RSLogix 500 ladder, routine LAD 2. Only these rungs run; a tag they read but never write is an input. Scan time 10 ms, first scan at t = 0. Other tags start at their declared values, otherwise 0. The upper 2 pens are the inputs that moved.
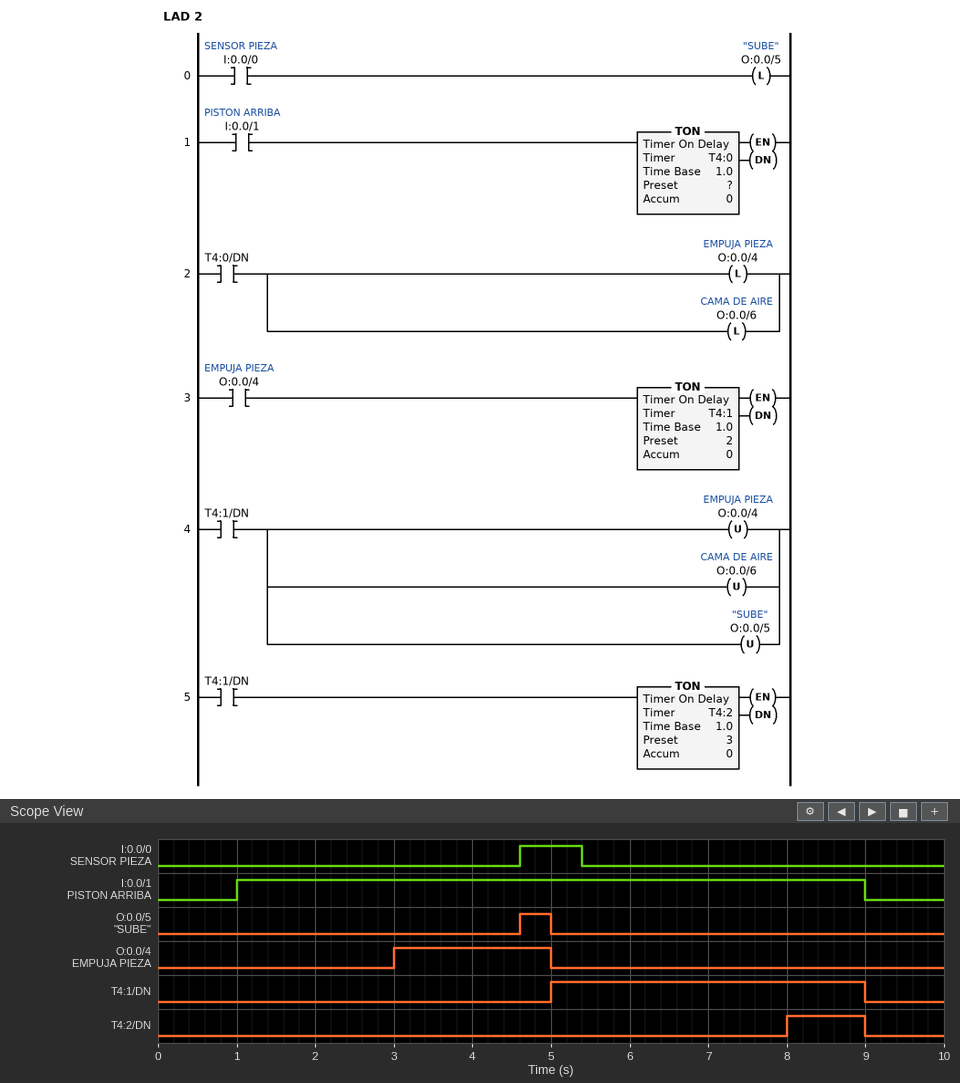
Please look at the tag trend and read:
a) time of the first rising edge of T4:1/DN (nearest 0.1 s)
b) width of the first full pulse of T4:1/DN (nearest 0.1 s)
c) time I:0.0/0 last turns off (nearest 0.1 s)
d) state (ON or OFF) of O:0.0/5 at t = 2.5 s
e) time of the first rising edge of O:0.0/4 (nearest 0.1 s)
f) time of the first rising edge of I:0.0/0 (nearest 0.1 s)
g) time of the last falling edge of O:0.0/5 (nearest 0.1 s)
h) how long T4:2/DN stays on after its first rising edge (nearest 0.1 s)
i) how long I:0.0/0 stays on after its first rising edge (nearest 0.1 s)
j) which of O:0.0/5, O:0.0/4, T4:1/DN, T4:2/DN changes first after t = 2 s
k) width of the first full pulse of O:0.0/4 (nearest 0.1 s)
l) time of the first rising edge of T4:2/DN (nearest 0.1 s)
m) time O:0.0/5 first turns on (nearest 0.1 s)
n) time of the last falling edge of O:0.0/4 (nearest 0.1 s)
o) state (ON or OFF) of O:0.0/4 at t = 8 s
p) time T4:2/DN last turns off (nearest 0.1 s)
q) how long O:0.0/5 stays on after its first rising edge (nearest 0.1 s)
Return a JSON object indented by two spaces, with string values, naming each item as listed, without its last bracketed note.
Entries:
{
  "time of the first rising edge of T4:1/DN": "5.0 s",
  "width of the first full pulse of T4:1/DN": "4.0 s",
  "time I:0.0/0 last turns off": "5.4 s",
  "state (ON or OFF) of O:0.0/5 at t = 2.5 s": "OFF",
  "time of the first rising edge of O:0.0/4": "3.0 s",
  "time of the first rising edge of I:0.0/0": "4.6 s",
  "time of the last falling edge of O:0.0/5": "5.0 s",
  "how long T4:2/DN stays on after its first rising edge": "1.0 s",
  "how long I:0.0/0 stays on after its first rising edge": "0.8 s",
  "which of O:0.0/5, O:0.0/4, T4:1/DN, T4:2/DN changes first after t = 2 s": "O:0.0/4",
  "width of the first full pulse of O:0.0/4": "2.0 s",
  "time of the first rising edge of T4:2/DN": "8.0 s",
  "time O:0.0/5 first turns on": "4.6 s",
  "time of the last falling edge of O:0.0/4": "5.0 s",
  "state (ON or OFF) of O:0.0/4 at t = 8 s": "OFF",
  "time T4:2/DN last turns off": "9.0 s",
  "how long O:0.0/5 stays on after its first rising edge": "0.4 s"
}
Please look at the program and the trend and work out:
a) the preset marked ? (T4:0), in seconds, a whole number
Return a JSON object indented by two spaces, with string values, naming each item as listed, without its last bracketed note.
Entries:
{
  "the preset marked ? (T4:0), in seconds, a whole number": "2 s"
}
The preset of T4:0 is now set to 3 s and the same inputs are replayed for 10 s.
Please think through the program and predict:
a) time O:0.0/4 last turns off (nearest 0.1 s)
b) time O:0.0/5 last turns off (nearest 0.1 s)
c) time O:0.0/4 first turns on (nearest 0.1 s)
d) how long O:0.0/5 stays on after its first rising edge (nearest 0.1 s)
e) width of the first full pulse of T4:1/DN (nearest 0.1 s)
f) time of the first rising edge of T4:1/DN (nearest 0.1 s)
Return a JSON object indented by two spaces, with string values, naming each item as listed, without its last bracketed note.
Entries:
{
  "time O:0.0/4 last turns off": "6.0 s",
  "time O:0.0/5 last turns off": "6.0 s",
  "time O:0.0/4 first turns on": "4.0 s",
  "how long O:0.0/5 stays on after its first rising edge": "1.4 s",
  "width of the first full pulse of T4:1/DN": "3.0 s",
  "time of the first rising edge of T4:1/DN": "6.0 s"
}
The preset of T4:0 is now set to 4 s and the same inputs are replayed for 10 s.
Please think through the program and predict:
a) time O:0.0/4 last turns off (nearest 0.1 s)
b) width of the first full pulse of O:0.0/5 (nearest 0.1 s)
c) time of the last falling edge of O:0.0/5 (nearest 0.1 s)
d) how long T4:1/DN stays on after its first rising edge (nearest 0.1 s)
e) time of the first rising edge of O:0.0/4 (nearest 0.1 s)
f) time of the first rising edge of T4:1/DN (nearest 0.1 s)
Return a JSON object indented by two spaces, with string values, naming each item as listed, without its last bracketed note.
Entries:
{
  "time O:0.0/4 last turns off": "7.0 s",
  "width of the first full pulse of O:0.0/5": "2.4 s",
  "time of the last falling edge of O:0.0/5": "7.0 s",
  "how long T4:1/DN stays on after its first rising edge": "2.0 s",
  "time of the first rising edge of O:0.0/4": "5.0 s",
  "time of the first rising edge of T4:1/DN": "7.0 s"
}
